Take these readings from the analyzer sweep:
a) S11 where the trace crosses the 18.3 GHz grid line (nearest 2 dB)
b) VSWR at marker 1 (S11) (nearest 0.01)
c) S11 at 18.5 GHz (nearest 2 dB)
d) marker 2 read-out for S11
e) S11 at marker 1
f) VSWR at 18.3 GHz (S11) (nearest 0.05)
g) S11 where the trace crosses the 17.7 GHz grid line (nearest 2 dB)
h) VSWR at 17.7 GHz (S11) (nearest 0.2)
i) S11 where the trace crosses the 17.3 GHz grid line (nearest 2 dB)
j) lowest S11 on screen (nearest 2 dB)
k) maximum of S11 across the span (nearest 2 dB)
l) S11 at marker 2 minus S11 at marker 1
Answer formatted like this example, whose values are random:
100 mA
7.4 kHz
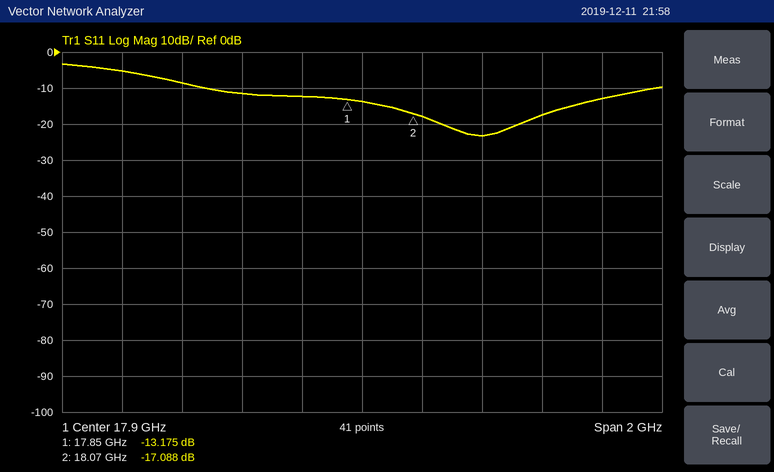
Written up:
-24 dB
1.56
-18 dB
-17.088 dB
-13.175 dB
1.15
-12 dB
1.6
-8 dB
-24 dB
-4 dB
-3.913 dB
